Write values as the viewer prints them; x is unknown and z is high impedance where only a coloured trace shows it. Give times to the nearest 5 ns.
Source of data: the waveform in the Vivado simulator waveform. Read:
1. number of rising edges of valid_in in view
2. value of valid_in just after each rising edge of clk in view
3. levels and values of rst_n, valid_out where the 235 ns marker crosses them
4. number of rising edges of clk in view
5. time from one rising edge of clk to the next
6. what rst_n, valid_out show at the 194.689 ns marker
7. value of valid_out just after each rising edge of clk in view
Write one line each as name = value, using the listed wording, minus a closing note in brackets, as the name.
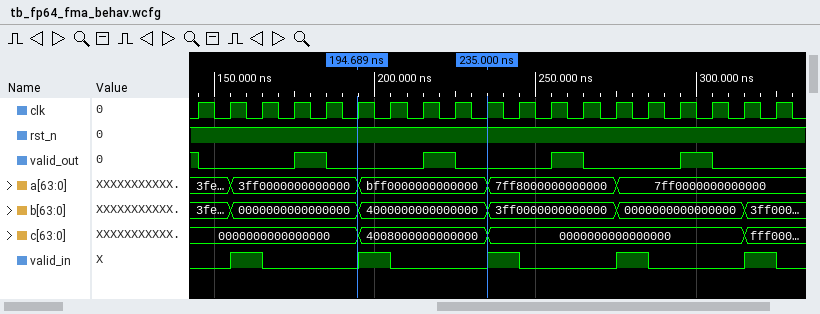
number of rising edges of valid_in in view = 5
value of valid_in just after each rising edge of clk in view = 0 1 0 0 0 1 0 0 0 1 0 0 0 1 0 0 0 1 0
levels and values of rst_n, valid_out where the 235 ns marker crosses them = rst_n=1, valid_out=0
number of rising edges of clk in view = 19
time from one rising edge of clk to the next = 10 ns
what rst_n, valid_out show at the 194.689 ns marker = rst_n=1, valid_out=0
value of valid_out just after each rising edge of clk in view = 0 0 0 1 0 0 0 1 0 0 0 1 0 0 0 1 0 0 0
